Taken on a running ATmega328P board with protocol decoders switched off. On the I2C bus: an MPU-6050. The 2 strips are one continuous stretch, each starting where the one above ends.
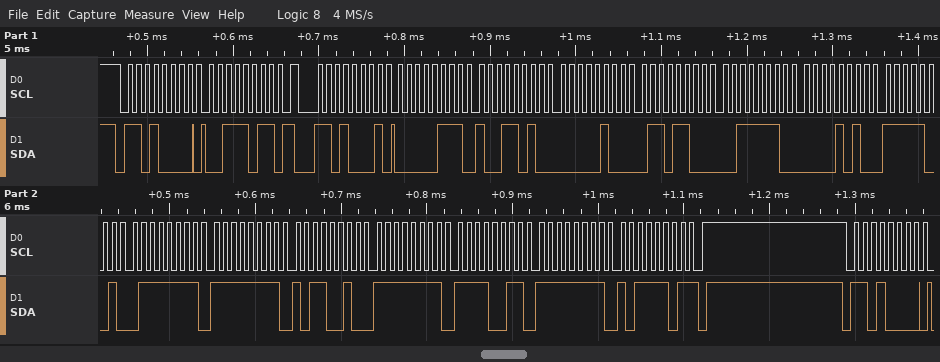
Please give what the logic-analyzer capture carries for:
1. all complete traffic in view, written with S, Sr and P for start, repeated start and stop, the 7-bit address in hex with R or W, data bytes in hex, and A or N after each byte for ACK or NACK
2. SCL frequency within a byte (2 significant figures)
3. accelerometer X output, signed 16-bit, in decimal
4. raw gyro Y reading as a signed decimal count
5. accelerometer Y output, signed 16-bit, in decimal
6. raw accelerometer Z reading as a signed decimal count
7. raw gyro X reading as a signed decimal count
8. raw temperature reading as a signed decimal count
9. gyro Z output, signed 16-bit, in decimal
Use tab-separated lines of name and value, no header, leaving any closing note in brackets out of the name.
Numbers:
all complete traffic in view, written with S, Sr and P for start, repeated start and stop, the 7-bit address in hex with R or W, data bytes in hex, and A or N after each byte for ACK or NACK	S 68W A 3B A Sr 68R A 07 A 9A A 04 A 6C A 3E A 0A A F9 A 7F A FF A B2 A FF A F3 A FF A BD N P S 68W A
SCL frequency within a byte	100 kHz
accelerometer X output, signed 16-bit, in decimal	1946
raw gyro Y reading as a signed decimal count	-13
accelerometer Y output, signed 16-bit, in decimal	1132
raw accelerometer Z reading as a signed decimal count	15882
raw gyro X reading as a signed decimal count	-78
raw temperature reading as a signed decimal count	-1665
gyro Z output, signed 16-bit, in decimal	-67
